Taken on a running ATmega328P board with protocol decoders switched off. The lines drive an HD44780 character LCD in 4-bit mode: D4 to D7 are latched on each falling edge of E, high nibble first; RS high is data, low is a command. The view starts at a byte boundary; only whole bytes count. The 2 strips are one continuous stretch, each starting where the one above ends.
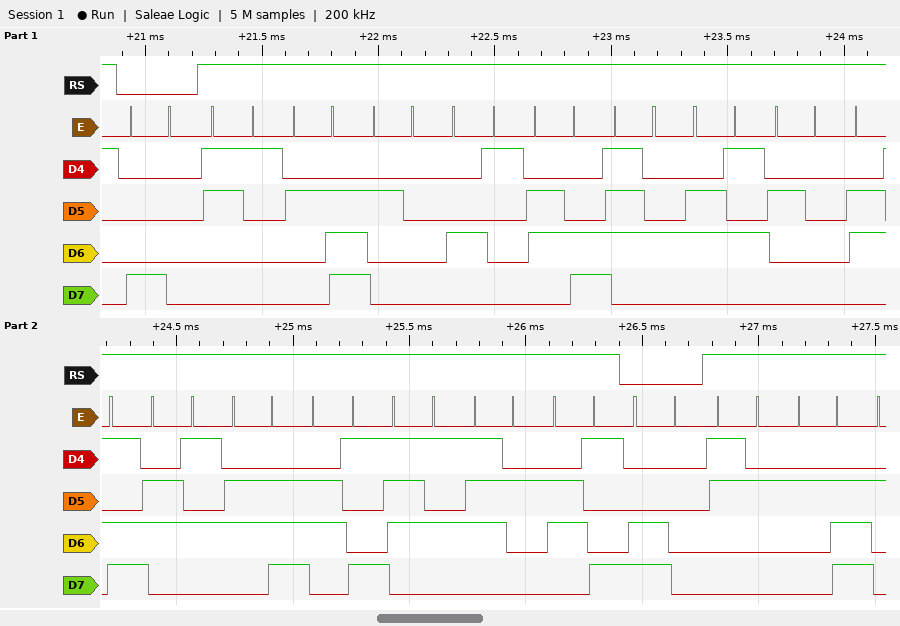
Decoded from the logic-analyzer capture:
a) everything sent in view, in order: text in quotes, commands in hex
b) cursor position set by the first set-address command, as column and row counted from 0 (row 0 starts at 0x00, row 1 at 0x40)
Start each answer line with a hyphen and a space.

- 0x80 "1. Alte meniuri" 0xC0 "2."
- column 0, row 0
